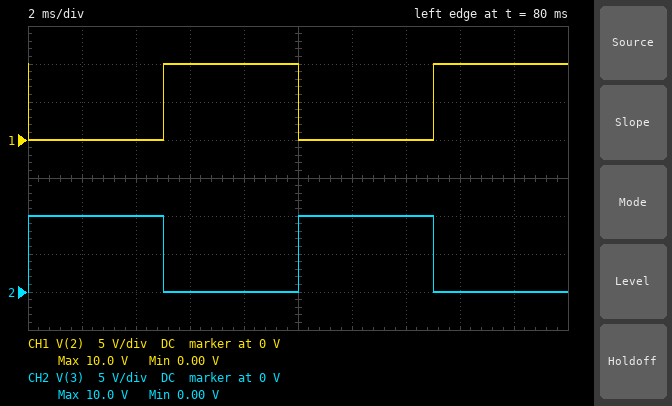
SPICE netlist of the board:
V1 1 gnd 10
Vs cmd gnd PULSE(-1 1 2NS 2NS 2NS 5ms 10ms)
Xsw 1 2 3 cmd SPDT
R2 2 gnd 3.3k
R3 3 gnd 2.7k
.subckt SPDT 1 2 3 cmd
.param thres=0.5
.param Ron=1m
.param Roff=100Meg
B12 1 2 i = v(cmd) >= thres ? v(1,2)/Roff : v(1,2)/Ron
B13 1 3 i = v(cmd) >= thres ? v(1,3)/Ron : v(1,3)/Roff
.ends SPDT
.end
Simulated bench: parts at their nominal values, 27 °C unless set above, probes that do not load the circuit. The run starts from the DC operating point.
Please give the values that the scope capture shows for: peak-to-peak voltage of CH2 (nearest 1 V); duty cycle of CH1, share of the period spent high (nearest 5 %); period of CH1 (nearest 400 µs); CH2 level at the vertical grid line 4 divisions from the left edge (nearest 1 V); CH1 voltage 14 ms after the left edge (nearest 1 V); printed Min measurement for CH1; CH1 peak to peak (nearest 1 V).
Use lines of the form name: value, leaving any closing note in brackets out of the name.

peak-to-peak voltage of CH2: 10 V
duty cycle of CH1, share of the period spent high: 50 %
period of CH1: 10.0 ms
CH2 level at the vertical grid line 4 divisions from the left edge: 0 V
CH1 voltage 14 ms after the left edge: 0 V
printed Min measurement for CH1: 0.00 V
CH1 peak to peak: 10 V
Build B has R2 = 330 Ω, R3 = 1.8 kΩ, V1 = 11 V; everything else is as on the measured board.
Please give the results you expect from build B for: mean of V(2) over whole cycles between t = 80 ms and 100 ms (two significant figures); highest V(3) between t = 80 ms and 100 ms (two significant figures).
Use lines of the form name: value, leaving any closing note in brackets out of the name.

mean of V(2) over whole cycles between t = 80 ms and 100 ms: 5.5 V
highest V(3) between t = 80 ms and 100 ms: 11 V
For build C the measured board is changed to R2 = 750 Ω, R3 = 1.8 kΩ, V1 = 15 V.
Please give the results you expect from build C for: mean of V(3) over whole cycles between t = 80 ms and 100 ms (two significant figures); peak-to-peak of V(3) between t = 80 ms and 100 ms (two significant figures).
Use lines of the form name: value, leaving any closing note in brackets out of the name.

mean of V(3) over whole cycles between t = 80 ms and 100 ms: 7.5 V
peak-to-peak of V(3) between t = 80 ms and 100 ms: 15 V
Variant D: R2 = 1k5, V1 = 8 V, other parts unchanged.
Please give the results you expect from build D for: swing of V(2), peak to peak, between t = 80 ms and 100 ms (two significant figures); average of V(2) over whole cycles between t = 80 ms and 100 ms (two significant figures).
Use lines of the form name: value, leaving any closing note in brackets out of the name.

swing of V(2), peak to peak, between t = 80 ms and 100 ms: 8.0 V
average of V(2) over whole cycles between t = 80 ms and 100 ms: 4.0 V
